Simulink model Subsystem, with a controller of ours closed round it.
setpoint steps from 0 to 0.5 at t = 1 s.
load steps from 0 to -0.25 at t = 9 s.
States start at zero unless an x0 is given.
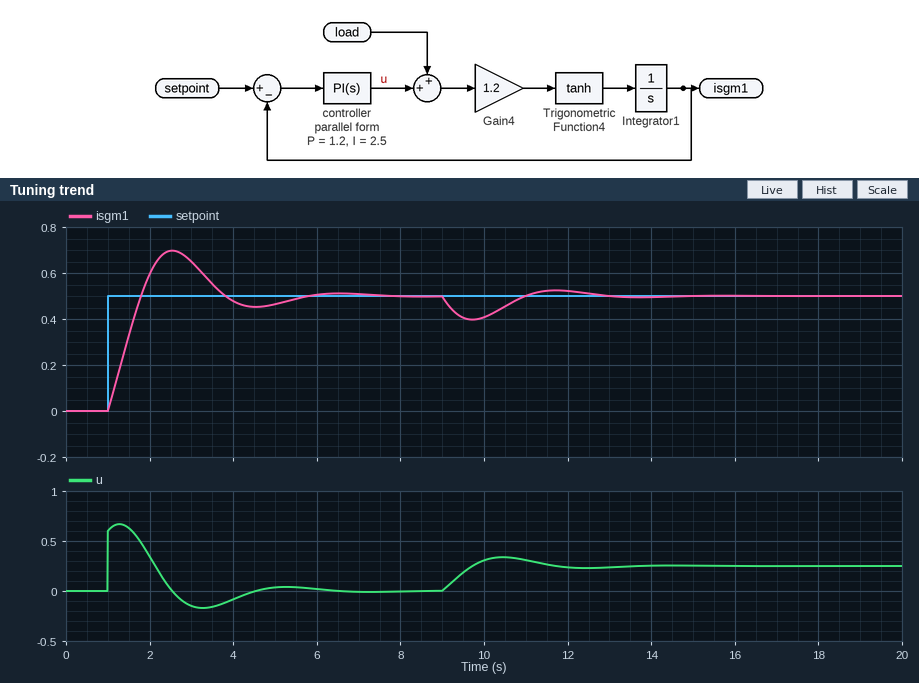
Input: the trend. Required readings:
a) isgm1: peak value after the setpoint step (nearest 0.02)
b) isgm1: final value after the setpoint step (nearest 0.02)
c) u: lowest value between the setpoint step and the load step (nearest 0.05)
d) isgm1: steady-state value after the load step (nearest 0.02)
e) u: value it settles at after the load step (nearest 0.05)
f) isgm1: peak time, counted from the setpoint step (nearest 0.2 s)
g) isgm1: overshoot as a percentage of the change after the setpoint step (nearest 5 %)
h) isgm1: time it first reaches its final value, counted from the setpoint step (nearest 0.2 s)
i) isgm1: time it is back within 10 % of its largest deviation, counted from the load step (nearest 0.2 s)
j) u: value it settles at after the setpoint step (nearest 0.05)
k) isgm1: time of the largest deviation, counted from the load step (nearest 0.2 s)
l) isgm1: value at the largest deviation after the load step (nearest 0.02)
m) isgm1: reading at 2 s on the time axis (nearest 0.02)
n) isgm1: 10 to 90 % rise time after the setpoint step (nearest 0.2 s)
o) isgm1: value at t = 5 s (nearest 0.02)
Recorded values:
0.70
0.50
-0.15
0.50
0.25
1.6 s
40 %
0.8 s
3.6 s
0.00
0.8 s
0.40
0.60
0.6 s
0.46
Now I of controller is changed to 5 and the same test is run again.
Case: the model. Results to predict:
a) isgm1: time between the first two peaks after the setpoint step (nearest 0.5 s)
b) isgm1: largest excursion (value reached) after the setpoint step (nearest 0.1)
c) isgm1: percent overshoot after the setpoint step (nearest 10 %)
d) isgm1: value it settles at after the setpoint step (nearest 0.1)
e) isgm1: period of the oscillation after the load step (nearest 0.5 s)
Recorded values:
2.5 s
0.8
50 %
0.5
2.5 s
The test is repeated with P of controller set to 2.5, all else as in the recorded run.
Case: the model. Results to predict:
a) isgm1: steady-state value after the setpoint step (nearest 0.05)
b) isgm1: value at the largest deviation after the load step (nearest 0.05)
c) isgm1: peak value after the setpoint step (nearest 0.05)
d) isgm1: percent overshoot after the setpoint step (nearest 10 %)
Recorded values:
0.50
0.45
0.60
20 %
